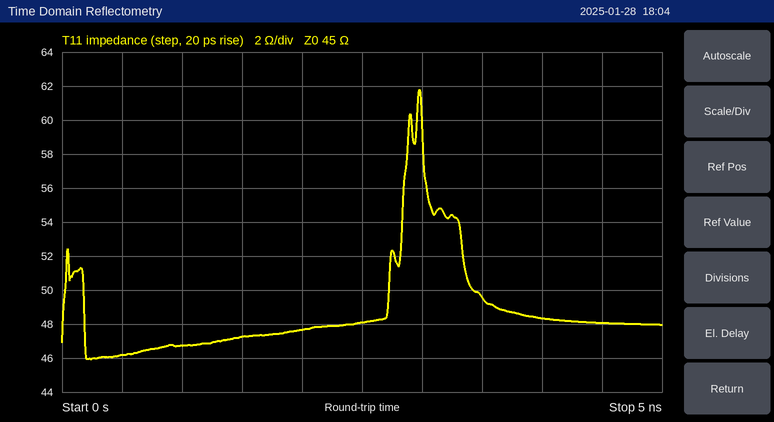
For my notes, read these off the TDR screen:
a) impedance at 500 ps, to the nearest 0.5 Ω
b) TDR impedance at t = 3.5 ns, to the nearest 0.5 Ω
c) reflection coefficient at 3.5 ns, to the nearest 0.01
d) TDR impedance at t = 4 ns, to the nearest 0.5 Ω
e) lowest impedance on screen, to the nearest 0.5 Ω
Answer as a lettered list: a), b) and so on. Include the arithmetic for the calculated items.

a) 46.0 Ω
b) 49.5 Ω
c) (49.5 − 45)/(49.5 + 45) ≈ +0.05
d) 48.5 Ω
e) 46.0 Ω
